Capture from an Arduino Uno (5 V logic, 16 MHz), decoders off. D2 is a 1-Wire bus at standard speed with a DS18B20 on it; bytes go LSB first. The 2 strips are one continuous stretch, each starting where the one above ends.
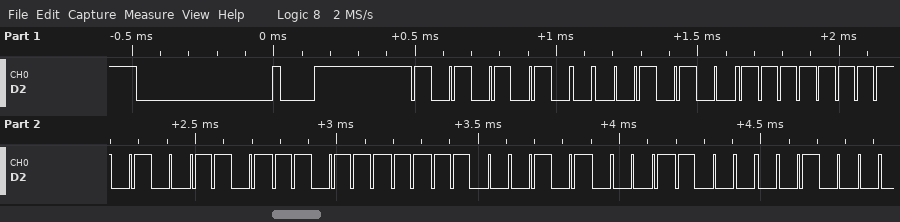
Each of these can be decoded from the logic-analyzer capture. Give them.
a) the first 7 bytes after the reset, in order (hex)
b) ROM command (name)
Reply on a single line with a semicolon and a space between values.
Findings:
55 28 FF B2 FB A3 18; Match ROM
